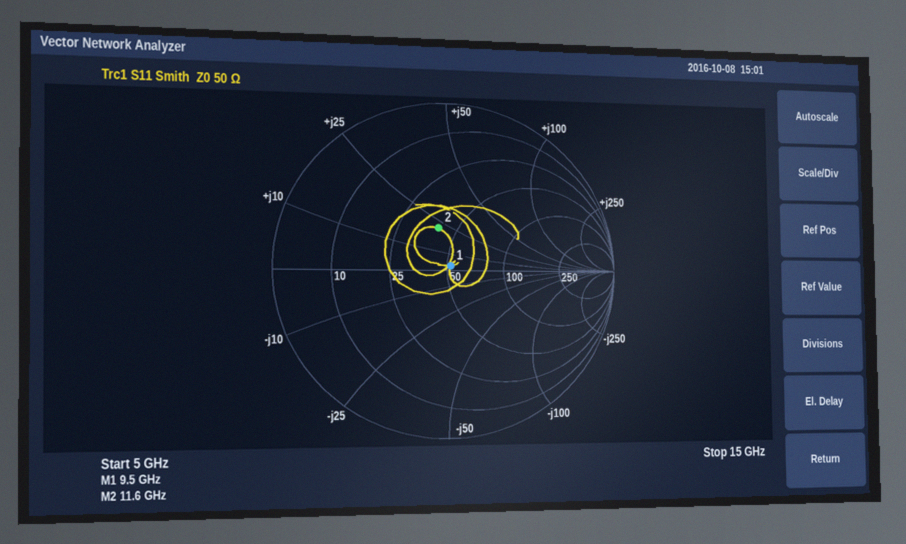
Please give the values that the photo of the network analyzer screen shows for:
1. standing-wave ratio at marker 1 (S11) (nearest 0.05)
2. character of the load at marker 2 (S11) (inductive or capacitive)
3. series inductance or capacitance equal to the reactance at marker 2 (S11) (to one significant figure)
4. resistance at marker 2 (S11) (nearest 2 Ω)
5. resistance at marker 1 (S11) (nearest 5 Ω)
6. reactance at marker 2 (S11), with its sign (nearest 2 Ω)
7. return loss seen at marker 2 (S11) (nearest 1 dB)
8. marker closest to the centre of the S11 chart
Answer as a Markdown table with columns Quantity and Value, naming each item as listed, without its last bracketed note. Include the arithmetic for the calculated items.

| Quantity | Value |
|---|---|
| standing-wave ratio at marker 1 (S11) | 1.05 |
| character of the load at marker 2 (S11) | inductive |
| series inductance or capacitance equal to the reactance at marker 2 (S11) | L = 22 Ω/(2π × 11.6 GHz) ≈ 302 pH, so 300 pH to one significant figure |
| resistance at marker 2 (S11) | 40 Ω |
| resistance at marker 1 (S11) | 50 Ω |
| reactance at marker 2 (S11), with its sign | +22 Ω |
| return loss seen at marker 2 (S11) | 12 dB |
| marker closest to the centre of the S11 chart | marker 1 |
